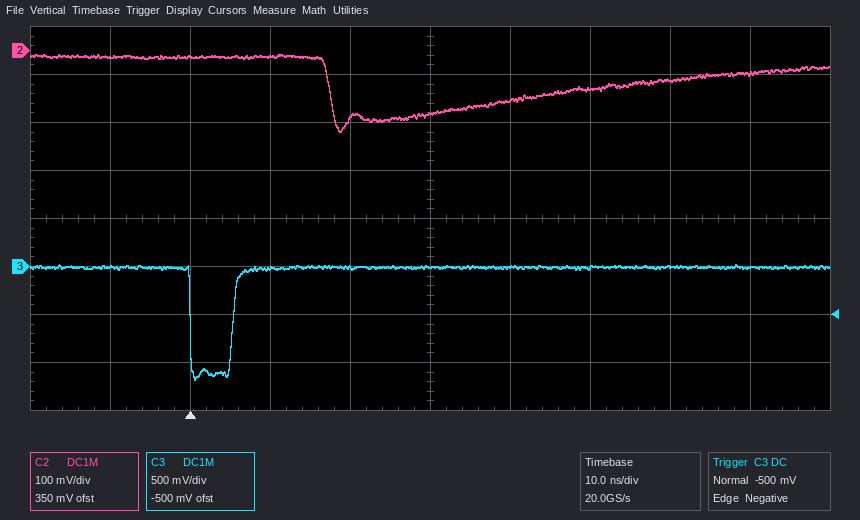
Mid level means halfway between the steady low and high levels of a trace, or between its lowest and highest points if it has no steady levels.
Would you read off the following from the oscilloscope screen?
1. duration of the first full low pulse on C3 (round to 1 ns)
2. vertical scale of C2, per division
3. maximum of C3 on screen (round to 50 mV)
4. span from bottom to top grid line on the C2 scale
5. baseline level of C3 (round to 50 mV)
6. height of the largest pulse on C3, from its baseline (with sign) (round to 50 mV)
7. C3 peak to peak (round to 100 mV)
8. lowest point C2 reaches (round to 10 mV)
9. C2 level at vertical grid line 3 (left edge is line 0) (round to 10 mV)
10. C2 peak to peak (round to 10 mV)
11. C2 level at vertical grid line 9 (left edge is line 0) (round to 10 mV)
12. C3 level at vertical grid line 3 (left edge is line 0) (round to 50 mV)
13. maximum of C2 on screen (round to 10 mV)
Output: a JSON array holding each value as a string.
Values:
["5 ns", "100 mV", "0 mV", "800 mV", "0 mV", "-1.15 V", "1.20 V", "-170 mV", "-10 mV", "160 mV", "-50 mV", "0 mV", "-10 mV"]
